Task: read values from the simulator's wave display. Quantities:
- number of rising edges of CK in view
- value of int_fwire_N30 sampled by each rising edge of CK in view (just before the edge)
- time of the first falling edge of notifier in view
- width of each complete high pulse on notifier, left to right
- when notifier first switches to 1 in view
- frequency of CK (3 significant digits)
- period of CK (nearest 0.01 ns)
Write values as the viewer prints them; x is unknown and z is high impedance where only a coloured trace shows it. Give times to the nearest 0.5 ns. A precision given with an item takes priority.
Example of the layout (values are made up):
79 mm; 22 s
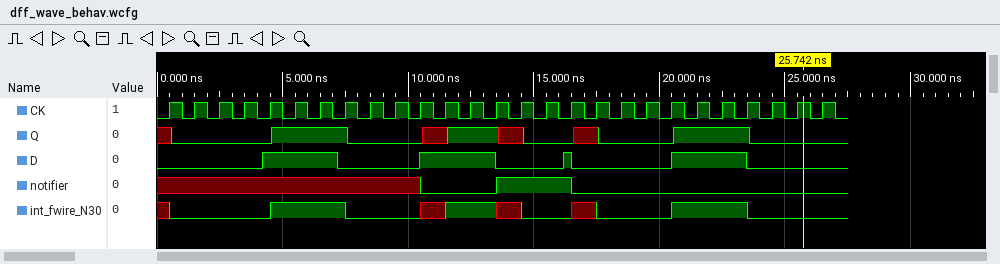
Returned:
27; x 0 0 0 0 1 1 1 0 0 0 x 1 1 x 0 0 x 0 0 0 1 1 1 0 0 0; 16.5 ns; 3 ns; 13.5 ns; 1.00 GHz; 1 ns
